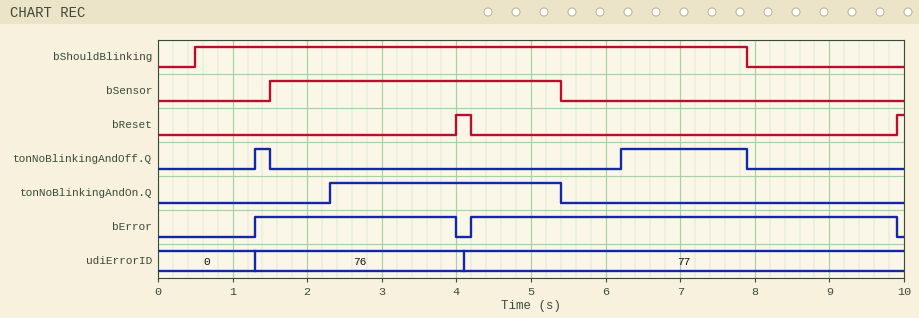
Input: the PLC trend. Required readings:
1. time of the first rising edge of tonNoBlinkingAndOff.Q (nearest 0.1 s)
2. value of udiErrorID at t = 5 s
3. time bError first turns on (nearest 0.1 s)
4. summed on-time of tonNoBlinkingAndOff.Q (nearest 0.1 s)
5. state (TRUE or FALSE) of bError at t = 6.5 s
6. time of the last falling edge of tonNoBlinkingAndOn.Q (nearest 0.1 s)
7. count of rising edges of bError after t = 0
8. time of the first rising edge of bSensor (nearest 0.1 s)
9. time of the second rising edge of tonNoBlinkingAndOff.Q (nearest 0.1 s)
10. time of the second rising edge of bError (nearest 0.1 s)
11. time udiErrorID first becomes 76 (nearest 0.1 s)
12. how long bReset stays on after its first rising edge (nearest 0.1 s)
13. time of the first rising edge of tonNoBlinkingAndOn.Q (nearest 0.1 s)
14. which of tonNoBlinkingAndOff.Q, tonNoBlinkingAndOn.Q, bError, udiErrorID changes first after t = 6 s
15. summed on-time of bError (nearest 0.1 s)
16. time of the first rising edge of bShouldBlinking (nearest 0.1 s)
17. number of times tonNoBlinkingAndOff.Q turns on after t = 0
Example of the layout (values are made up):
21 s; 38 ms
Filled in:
1.3 s; 77; 1.3 s; 1.9 s; TRUE; 5.4 s; 2; 1.5 s; 6.2 s; 4.2 s; 1.3 s; 0.2 s; 2.3 s; tonNoBlinkingAndOff.Q; 8.4 s; 0.5 s; 2
